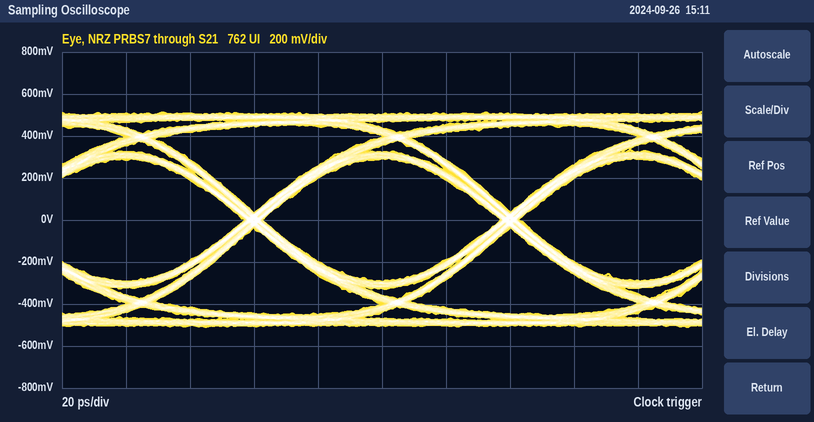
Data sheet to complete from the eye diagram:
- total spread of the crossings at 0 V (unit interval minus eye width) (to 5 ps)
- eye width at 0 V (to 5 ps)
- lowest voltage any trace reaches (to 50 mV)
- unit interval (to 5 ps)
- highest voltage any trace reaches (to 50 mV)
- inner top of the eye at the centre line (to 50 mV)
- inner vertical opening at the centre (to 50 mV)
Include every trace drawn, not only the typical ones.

5 ps
75 ps
-500 mV
80 ps
500 mV
300 mV
600 mV
